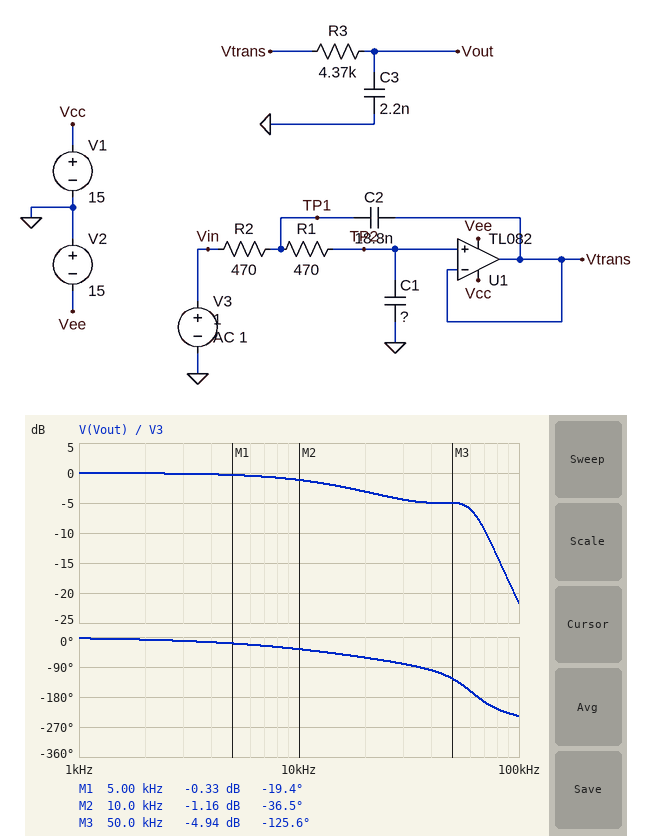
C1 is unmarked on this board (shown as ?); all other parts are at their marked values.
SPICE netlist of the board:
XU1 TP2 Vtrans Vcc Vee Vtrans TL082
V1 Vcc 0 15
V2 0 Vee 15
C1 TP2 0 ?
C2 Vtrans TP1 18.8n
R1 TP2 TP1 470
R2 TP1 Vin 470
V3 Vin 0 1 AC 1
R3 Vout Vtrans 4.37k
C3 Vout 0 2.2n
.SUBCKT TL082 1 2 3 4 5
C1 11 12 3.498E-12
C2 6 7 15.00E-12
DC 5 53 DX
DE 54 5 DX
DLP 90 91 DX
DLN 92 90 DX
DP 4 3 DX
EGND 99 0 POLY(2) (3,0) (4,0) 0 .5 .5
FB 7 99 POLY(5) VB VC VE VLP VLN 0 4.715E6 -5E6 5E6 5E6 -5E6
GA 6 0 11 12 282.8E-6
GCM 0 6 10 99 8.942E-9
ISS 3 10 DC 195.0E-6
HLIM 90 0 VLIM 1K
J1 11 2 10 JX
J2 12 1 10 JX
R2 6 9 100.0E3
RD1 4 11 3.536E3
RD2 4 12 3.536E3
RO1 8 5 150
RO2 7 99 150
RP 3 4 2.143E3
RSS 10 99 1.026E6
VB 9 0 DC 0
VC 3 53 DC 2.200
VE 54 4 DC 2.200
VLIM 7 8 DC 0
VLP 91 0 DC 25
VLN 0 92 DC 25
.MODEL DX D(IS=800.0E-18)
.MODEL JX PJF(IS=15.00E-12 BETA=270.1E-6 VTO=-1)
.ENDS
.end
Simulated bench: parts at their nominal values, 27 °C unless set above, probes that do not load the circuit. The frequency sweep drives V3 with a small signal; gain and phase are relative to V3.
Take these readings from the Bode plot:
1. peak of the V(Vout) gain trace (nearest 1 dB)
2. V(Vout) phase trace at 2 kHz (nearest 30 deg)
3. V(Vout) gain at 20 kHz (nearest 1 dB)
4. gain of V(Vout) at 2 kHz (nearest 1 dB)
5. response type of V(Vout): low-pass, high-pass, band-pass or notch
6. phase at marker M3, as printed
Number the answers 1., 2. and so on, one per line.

1. 0 dB
2. 0 deg
3. -3 dB
4. 0 dB
5. low-pass
6. -125.6 deg
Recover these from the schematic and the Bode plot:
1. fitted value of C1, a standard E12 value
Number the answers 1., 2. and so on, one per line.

1. 1.5 nF
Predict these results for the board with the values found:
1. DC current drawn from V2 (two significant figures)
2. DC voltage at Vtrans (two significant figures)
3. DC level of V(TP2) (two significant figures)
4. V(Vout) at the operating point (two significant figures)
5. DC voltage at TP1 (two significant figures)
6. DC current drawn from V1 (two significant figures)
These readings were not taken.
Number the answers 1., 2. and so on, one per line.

1. 14 mA
2. 1.0 V
3. 1.0 V
4. 1.0 V
5. 1.0 V
6. 14 mA
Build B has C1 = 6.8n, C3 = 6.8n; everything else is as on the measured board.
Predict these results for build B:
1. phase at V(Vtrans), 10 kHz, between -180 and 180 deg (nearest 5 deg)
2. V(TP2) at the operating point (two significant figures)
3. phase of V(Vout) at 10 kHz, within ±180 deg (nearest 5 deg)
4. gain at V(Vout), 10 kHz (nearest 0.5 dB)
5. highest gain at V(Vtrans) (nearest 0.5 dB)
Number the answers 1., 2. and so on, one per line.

1. -25 deg
2. 1.0 V
3. -85 deg
4. -6.5 dB
5. 0.5 dB
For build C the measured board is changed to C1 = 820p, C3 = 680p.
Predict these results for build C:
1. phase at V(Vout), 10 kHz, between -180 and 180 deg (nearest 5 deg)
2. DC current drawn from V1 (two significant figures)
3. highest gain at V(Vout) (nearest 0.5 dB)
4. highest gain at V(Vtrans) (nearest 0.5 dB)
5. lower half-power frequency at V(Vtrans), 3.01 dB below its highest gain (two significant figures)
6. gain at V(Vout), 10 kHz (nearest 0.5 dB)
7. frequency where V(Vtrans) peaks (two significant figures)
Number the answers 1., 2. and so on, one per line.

1. -15 deg
2. 14 mA
3. 3.5 dB
4. 8.5 dB
5. 60 kHz
6. 0 dB
7. 77 kHz
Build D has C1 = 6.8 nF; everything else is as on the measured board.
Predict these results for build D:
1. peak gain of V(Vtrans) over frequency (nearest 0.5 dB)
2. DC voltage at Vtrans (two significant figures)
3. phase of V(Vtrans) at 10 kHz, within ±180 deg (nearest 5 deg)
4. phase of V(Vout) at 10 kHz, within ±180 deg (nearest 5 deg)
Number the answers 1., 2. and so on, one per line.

1. 0.5 dB
2. 1.0 V
3. -25 deg
4. -55 deg
